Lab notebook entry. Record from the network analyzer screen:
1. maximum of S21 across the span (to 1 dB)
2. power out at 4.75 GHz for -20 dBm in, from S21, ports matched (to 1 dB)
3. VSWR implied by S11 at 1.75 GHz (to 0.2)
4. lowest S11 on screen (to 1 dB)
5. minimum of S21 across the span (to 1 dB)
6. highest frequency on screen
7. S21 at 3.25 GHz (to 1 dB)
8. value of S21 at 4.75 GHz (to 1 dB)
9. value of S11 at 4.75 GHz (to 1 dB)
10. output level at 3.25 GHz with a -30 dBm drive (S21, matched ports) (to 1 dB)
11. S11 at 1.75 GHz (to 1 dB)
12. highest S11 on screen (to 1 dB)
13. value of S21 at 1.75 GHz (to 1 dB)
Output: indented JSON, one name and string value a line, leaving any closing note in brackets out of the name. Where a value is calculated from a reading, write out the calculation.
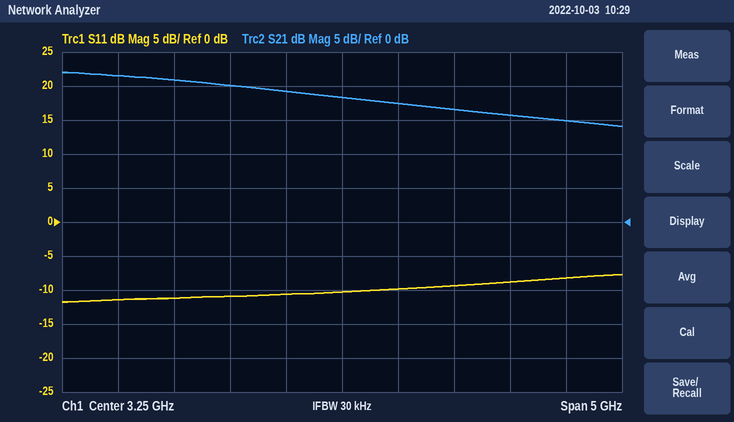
{
  "maximum of S21 across the span": "22 dB",
  "power out at 4.75 GHz for -20 dBm in, from S21, ports matched": "-20 dBm + (16 dB) = -4 dBm",
  "VSWR implied by S11 at 1.75 GHz": "|Γ| = 10^(-11/20) = 0.2818; VSWR = (1 + 0.2818)/(1 − 0.2818) ≈ 1.8",
  "lowest S11 on screen": "-12 dB",
  "minimum of S21 across the span": "14 dB",
  "highest frequency on screen": "5.75 GHz",
  "S21 at 3.25 GHz": "18 dB",
  "value of S21 at 4.75 GHz": "16 dB",
  "value of S11 at 4.75 GHz": "-9 dB",
  "output level at 3.25 GHz with a -30 dBm drive (S21, matched ports)": "-30 dBm + (18 dB) = -12 dBm",
  "S11 at 1.75 GHz": "-11 dB",
  "highest S11 on screen": "-8 dB",
  "value of S21 at 1.75 GHz": "21 dB"
}
